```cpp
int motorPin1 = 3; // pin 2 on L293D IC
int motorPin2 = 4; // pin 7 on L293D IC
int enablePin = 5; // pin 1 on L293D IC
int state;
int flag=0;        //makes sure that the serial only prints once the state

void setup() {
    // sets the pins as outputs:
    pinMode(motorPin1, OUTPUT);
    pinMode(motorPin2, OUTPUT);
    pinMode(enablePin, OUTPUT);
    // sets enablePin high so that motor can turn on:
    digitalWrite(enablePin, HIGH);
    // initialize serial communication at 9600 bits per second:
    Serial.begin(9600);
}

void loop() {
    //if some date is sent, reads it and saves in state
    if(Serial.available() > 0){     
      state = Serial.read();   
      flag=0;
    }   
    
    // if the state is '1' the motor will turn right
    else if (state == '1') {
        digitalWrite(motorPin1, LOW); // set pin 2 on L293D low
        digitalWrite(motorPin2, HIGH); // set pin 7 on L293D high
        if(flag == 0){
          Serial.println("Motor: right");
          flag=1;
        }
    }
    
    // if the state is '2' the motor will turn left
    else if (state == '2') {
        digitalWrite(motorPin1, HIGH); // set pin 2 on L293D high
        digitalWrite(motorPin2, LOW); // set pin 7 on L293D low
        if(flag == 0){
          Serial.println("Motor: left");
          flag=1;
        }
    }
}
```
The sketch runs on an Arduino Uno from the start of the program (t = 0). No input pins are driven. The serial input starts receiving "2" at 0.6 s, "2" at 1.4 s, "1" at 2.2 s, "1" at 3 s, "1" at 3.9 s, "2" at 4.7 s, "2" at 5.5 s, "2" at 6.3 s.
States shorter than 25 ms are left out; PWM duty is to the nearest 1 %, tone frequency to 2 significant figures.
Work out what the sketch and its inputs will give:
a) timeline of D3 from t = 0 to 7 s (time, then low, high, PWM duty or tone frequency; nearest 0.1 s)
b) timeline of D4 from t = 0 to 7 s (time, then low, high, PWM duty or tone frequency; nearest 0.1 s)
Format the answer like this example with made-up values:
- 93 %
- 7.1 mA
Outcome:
- 0 s low; 0.6 s high; 2.2 s low; 4.7 s high
- 0 s low; 2.2 s high; 4.7 s low
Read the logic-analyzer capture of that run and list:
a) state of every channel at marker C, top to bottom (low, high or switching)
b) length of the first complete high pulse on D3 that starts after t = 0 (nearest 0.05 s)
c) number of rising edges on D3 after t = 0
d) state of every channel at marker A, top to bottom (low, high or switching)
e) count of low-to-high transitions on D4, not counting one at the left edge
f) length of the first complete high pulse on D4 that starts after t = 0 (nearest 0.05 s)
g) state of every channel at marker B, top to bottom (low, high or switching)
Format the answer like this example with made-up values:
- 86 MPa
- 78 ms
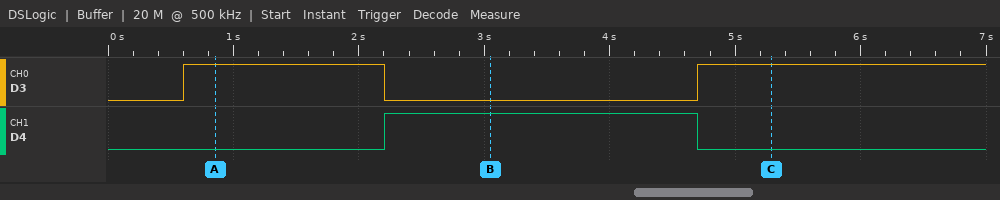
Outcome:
- D3 high, D4 low
- 1.60 s
- 2
- D3 high, D4 low
- 1
- 2.50 s
- D3 low, D4 high
